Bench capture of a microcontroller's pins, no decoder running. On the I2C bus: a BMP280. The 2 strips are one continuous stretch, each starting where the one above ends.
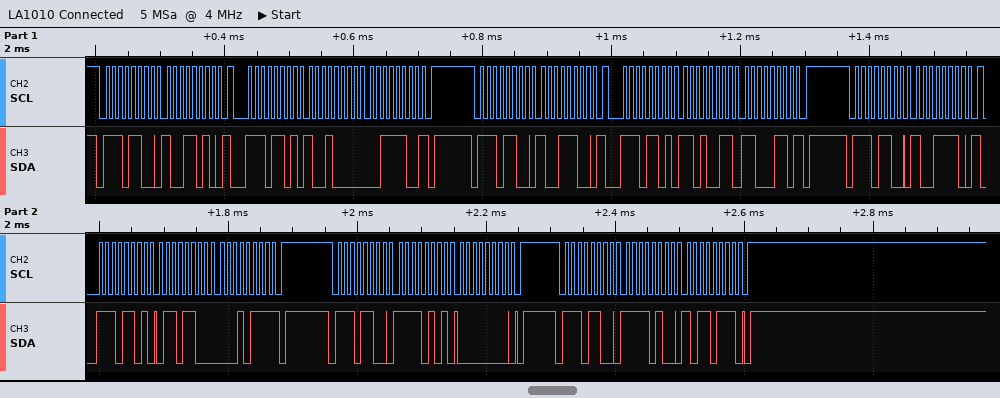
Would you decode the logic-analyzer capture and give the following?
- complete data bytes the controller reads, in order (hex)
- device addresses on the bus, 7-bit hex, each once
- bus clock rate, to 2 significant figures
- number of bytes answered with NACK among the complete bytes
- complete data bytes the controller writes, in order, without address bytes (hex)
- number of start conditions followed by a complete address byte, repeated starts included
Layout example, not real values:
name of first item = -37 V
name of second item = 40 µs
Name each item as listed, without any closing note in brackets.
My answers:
complete data bytes the controller reads, in order = 90 3C D3 C6 6C 17
device addresses on the bus, 7-bit hex, each once = 0x76
bus clock rate, to 2 significant figures = 100 kHz
number of bytes answered with NACK among the complete bytes = 3
complete data bytes the controller writes, in order, without address bytes = 9A 9C 9E F5 00 F4 B7
number of start conditions followed by a complete address byte, repeated starts included = 8
